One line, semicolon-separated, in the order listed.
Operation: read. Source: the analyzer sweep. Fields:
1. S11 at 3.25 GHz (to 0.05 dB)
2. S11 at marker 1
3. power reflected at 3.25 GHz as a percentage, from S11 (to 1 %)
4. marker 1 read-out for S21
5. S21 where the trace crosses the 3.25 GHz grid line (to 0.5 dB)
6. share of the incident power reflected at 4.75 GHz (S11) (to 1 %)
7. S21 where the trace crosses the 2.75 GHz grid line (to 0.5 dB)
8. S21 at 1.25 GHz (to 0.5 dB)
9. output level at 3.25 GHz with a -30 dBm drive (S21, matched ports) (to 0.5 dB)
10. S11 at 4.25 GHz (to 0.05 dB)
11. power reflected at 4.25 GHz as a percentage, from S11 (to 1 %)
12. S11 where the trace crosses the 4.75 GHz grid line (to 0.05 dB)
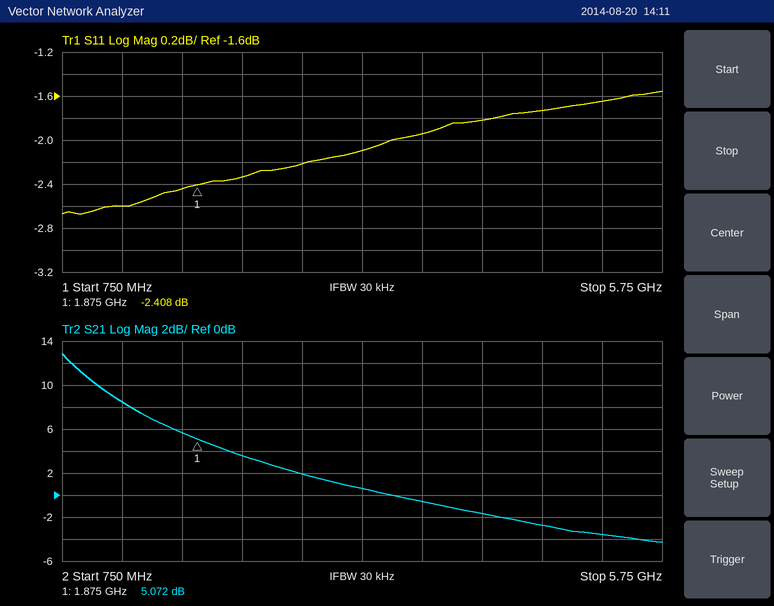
-2.10 dB; -2.408 dB; 62 %; 5.072 dB; 0.5 dB; 67 %; 2.0 dB; 8.5 dB; -29.5 dBm; -1.80 dB; 66 %; -1.75 dB
